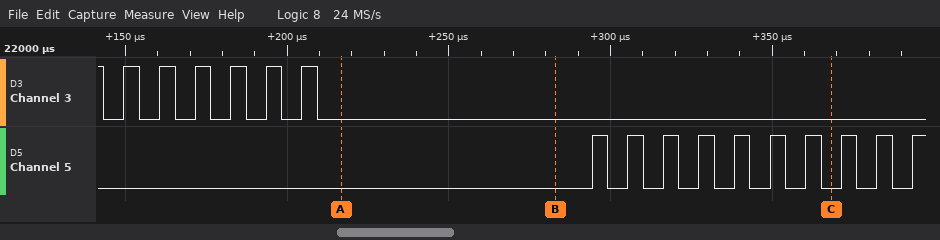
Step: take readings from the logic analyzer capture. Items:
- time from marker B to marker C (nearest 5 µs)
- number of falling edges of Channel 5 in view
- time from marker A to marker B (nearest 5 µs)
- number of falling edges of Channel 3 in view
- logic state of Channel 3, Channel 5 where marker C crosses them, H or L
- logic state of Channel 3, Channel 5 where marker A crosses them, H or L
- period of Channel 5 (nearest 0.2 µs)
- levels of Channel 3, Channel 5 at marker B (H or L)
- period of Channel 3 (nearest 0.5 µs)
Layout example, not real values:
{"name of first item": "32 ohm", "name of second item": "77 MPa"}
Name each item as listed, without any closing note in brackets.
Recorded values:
{"time from marker B to marker C": "85 µs", "number of falling edges of Channel 5 in view": "9", "time from marker A to marker B": "65 µs", "number of falling edges of Channel 3 in view": "7", "logic state of Channel 3, Channel 5 where marker C crosses them, H or L": "Channel 3=L, Channel 5=L", "logic state of Channel 3, Channel 5 where marker A crosses them, H or L": "Channel 3=L, Channel 5=L", "period of Channel 5": "11 µs", "levels of Channel 3, Channel 5 at marker B": "Channel 3=L, Channel 5=L", "period of Channel 3": "11 µs"}
